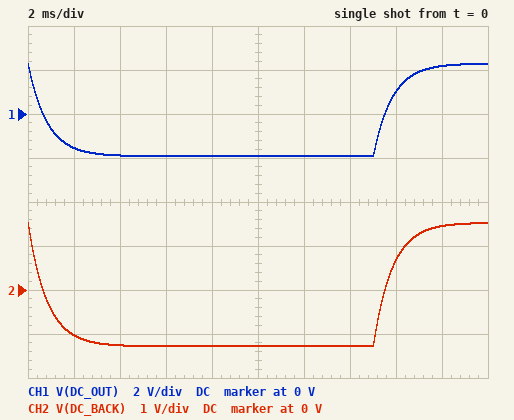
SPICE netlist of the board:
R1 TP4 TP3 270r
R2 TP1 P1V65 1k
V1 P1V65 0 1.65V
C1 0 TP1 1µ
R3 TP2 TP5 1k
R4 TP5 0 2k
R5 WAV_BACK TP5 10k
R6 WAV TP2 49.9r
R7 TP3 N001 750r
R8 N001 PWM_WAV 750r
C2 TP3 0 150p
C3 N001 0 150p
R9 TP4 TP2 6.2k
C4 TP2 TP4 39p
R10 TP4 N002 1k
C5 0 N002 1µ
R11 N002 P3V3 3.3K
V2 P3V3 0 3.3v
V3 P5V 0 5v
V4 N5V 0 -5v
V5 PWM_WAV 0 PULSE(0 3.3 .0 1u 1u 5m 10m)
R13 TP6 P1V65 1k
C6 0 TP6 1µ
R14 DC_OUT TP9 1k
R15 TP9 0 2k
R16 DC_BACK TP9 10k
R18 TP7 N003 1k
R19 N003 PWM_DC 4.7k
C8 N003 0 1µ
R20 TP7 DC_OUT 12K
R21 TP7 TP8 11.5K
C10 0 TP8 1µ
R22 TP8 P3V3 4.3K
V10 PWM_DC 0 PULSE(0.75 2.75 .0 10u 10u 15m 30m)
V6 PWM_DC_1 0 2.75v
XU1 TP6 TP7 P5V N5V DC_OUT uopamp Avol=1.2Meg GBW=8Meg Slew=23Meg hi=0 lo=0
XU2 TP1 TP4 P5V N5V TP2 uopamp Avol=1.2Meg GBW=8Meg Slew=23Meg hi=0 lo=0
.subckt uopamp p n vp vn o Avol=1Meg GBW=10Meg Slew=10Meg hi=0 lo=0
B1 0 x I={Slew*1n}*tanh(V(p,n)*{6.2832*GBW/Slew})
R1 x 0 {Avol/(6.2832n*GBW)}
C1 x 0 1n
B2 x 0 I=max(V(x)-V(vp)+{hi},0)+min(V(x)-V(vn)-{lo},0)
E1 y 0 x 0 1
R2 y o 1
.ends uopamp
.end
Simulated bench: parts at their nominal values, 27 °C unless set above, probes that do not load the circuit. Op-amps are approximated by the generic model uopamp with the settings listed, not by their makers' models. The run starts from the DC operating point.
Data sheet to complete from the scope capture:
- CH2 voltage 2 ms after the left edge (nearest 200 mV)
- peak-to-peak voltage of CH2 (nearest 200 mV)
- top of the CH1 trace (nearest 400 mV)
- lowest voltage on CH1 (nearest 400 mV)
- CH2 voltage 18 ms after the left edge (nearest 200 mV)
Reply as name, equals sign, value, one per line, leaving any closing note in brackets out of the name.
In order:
CH2 voltage 2 ms after the left edge = -1.0 V
peak-to-peak voltage of CH2 = 2.8 V
top of the CH1 trace = 2.4 V
lowest voltage on CH1 = -2.0 V
CH2 voltage 18 ms after the left edge = 1.4 V
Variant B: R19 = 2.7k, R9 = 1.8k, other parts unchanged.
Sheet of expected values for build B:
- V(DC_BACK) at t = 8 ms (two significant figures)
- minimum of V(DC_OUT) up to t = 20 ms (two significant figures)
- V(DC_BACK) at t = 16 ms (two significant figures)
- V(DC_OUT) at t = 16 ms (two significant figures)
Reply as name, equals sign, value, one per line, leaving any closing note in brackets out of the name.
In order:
V(DC_BACK) at t = 8 ms = -2.1 V
minimum of V(DC_OUT) up to t = 20 ms = -3.2 V
V(DC_BACK) at t = 16 ms = 1.1 V
V(DC_OUT) at t = 16 ms = 1.6 V
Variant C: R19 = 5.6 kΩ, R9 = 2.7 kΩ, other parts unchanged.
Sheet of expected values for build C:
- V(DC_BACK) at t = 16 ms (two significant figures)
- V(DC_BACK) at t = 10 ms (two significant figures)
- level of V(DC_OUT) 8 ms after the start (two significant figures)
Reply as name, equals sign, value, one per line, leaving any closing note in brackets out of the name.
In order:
V(DC_BACK) at t = 16 ms = 600 mV
V(DC_BACK) at t = 10 ms = -1.1 V
level of V(DC_OUT) 8 ms after the start = -1.6 V
